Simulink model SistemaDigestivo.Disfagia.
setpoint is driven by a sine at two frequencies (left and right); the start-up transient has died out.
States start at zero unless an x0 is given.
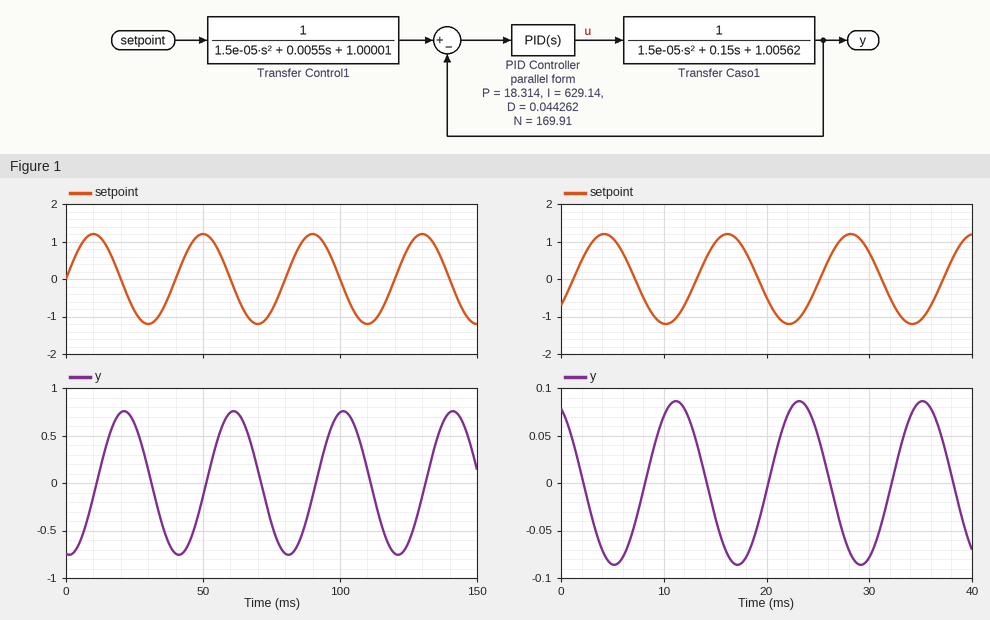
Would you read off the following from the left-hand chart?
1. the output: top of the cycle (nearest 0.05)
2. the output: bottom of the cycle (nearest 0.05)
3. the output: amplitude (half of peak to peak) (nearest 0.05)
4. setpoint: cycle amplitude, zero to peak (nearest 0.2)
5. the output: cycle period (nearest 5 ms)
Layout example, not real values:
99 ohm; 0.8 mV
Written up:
0.75; -0.75; 0.75; 1.2; 40 ms
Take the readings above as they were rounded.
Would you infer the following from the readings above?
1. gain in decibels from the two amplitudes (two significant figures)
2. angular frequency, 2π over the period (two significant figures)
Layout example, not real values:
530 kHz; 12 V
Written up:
-4.1 dB; 0.16 rad/ms
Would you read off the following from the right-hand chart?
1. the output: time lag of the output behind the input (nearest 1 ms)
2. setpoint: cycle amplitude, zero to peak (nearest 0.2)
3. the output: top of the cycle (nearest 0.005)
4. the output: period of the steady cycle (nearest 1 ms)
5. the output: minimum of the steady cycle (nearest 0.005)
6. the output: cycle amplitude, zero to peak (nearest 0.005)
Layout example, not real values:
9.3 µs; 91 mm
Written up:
7 ms; 1.2; 0.085; 12 ms; -0.085; 0.085
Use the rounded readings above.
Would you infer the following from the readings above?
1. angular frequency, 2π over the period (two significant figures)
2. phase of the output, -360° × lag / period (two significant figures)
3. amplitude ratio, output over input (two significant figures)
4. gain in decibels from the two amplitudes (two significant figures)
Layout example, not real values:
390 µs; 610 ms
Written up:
0.52 rad/ms; -210°; 0.071; -23 dB
